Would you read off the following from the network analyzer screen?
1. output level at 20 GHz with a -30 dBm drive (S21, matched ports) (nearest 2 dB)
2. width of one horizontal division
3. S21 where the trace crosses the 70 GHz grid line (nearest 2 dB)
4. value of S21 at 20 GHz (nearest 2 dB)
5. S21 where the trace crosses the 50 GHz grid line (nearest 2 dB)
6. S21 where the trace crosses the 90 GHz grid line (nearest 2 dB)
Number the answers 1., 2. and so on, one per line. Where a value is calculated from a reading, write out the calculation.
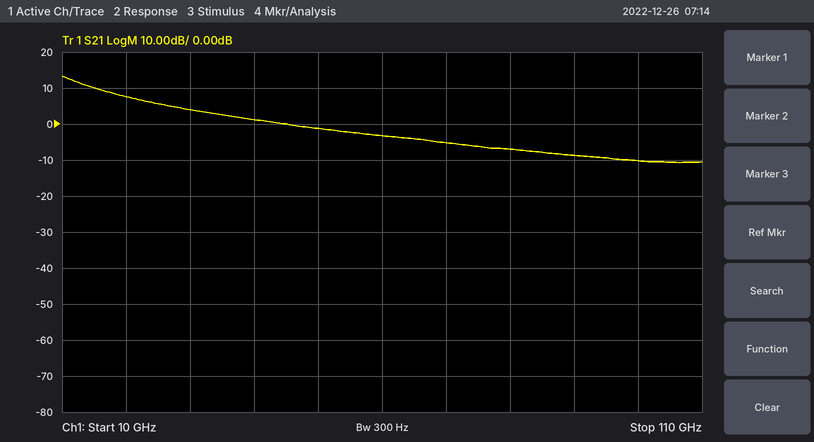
1. -30 dBm + (8 dB) = -22 dBm
2. 10 GHz
3. -6 dB
4. 8 dB
5. -2 dB
6. -8 dB
